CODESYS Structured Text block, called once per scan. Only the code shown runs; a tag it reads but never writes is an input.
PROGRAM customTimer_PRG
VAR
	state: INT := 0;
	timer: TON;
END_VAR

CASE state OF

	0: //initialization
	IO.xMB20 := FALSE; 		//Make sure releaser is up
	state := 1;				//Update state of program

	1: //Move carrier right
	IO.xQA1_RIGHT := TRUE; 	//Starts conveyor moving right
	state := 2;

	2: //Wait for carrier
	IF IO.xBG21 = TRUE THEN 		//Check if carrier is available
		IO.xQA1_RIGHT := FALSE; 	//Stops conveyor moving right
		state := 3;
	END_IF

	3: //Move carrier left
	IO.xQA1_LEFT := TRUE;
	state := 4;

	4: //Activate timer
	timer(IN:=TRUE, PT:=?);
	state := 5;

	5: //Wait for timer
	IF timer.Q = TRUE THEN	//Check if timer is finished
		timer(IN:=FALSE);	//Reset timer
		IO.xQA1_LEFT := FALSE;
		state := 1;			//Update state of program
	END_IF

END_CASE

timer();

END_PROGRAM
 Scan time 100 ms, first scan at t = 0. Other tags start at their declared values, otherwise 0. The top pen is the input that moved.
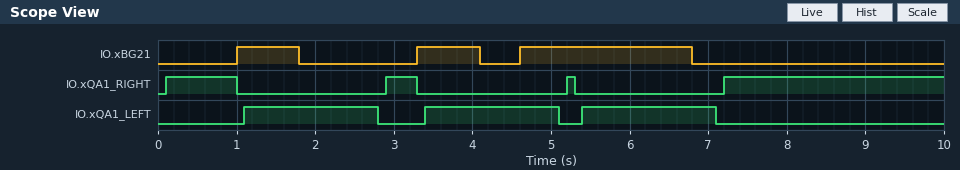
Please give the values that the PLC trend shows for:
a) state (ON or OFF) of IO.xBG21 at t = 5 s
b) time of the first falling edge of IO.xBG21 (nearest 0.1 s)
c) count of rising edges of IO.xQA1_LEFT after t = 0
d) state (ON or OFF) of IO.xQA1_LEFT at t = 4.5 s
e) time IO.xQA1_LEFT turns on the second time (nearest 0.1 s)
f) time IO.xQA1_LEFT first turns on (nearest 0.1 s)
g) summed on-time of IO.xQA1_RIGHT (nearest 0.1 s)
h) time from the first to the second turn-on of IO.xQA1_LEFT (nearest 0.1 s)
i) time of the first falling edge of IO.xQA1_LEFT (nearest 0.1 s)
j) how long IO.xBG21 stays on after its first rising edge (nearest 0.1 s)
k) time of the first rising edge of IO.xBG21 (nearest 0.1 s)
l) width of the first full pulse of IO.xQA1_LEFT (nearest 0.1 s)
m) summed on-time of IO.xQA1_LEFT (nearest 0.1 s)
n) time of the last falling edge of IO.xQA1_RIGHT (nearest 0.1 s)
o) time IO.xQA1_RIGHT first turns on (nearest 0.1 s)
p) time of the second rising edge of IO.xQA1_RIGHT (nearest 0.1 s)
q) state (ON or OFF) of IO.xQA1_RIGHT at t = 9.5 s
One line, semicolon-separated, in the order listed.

ON; 1.8 s; 3; ON; 3.4 s; 1.1 s; 4.2 s; 2.3 s; 2.8 s; 0.8 s; 1.0 s; 1.7 s; 5.1 s; 5.3 s; 0.1 s; 2.9 s; ON
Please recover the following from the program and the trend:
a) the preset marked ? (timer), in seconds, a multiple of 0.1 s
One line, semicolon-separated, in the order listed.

1.5 s
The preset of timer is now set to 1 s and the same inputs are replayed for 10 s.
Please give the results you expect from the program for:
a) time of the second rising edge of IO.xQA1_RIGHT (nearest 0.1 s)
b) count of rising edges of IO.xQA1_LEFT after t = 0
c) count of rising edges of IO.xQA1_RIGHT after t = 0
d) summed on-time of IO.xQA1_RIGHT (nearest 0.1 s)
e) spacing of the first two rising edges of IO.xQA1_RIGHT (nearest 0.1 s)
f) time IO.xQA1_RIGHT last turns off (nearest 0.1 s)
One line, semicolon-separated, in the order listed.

2.4 s; 4; 5; 4.3 s; 2.3 s; 6.3 s
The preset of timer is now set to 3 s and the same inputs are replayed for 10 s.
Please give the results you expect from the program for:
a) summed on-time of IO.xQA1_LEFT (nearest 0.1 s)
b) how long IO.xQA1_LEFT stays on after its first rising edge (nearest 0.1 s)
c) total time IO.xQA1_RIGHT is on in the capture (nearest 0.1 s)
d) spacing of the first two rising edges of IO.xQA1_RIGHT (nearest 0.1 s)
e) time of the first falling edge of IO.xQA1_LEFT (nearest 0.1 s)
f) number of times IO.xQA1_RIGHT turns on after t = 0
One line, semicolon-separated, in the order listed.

6.4 s; 3.2 s; 3.1 s; 4.3 s; 4.3 s; 3
